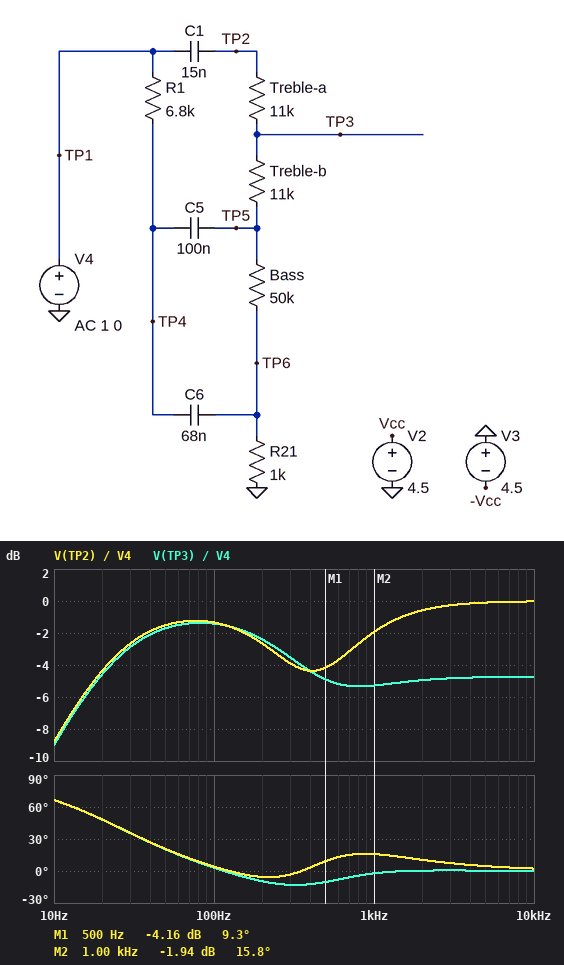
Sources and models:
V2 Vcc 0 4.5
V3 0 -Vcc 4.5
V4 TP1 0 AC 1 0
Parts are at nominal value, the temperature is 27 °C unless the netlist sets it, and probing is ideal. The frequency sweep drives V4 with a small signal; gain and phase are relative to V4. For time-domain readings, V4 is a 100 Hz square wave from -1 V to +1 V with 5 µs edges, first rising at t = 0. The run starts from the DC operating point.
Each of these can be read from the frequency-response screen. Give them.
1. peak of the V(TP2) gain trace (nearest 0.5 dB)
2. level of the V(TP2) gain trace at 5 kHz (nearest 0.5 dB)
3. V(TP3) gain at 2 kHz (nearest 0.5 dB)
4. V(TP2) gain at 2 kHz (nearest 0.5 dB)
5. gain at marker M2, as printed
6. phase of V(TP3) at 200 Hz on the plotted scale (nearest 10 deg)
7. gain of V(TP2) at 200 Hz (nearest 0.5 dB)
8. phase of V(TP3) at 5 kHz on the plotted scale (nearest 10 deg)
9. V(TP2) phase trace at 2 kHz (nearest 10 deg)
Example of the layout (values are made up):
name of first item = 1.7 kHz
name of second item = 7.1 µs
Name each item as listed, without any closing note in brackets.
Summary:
peak of the V(TP2) gain trace = 0 dB
level of the V(TP2) gain trace at 5 kHz = 0 dB
V(TP3) gain at 2 kHz = -5.0 dB
V(TP2) gain at 2 kHz = -0.5 dB
gain at marker M2, as printed = -1.94 dB
phase of V(TP3) at 200 Hz on the plotted scale = -10 deg
gain of V(TP2) at 200 Hz = -2.5 dB
phase of V(TP3) at 5 kHz on the plotted scale = 0 deg
V(TP2) phase trace at 2 kHz = 10 deg
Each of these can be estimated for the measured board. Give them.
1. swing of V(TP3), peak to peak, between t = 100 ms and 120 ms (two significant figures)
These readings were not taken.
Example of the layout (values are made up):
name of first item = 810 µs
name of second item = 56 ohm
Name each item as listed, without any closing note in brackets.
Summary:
swing of V(TP3), peak to peak, between t = 100 ms and 120 ms = 1.9 V
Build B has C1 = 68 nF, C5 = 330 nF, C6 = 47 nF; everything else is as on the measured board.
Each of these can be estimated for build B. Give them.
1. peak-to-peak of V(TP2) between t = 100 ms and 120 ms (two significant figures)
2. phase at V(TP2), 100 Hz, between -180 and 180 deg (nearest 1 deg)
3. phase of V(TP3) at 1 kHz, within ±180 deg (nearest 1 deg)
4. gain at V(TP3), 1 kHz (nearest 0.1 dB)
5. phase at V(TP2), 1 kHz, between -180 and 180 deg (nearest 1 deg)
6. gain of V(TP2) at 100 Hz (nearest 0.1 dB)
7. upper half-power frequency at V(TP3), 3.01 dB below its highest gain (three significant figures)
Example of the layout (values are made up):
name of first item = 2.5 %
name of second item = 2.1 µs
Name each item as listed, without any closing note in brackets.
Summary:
peak-to-peak of V(TP2) between t = 100 ms and 120 ms = 2.3 V
phase at V(TP2), 100 Hz, between -180 and 180 deg = 2 deg
phase of V(TP3) at 1 kHz, within ±180 deg = -11 deg
gain at V(TP3), 1 kHz = -3.3 dB
phase at V(TP2), 1 kHz, between -180 and 180 deg = 4 deg
gain of V(TP2) at 100 Hz = -0.8 dB
upper half-power frequency at V(TP3), 3.01 dB below its highest gain = 1.34 kHz
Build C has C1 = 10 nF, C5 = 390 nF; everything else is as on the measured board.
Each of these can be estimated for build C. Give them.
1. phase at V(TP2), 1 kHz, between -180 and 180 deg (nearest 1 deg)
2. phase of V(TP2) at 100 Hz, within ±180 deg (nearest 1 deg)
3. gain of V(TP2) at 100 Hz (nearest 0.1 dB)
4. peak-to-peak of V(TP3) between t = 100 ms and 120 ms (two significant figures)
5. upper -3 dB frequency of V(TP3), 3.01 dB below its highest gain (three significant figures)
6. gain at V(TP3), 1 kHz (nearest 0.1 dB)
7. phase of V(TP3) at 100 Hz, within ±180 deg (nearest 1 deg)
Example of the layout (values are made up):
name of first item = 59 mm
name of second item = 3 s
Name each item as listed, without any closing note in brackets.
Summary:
phase at V(TP2), 1 kHz, between -180 and 180 deg = 22 deg
phase of V(TP2) at 100 Hz, within ±180 deg = -7 deg
gain of V(TP2) at 100 Hz = -1.6 dB
peak-to-peak of V(TP3) between t = 100 ms and 120 ms = 1.8 V
upper -3 dB frequency of V(TP3), 3.01 dB below its highest gain = 292 Hz
gain at V(TP3), 1 kHz = -6.7 dB
phase of V(TP3) at 100 Hz, within ±180 deg = -8 deg
